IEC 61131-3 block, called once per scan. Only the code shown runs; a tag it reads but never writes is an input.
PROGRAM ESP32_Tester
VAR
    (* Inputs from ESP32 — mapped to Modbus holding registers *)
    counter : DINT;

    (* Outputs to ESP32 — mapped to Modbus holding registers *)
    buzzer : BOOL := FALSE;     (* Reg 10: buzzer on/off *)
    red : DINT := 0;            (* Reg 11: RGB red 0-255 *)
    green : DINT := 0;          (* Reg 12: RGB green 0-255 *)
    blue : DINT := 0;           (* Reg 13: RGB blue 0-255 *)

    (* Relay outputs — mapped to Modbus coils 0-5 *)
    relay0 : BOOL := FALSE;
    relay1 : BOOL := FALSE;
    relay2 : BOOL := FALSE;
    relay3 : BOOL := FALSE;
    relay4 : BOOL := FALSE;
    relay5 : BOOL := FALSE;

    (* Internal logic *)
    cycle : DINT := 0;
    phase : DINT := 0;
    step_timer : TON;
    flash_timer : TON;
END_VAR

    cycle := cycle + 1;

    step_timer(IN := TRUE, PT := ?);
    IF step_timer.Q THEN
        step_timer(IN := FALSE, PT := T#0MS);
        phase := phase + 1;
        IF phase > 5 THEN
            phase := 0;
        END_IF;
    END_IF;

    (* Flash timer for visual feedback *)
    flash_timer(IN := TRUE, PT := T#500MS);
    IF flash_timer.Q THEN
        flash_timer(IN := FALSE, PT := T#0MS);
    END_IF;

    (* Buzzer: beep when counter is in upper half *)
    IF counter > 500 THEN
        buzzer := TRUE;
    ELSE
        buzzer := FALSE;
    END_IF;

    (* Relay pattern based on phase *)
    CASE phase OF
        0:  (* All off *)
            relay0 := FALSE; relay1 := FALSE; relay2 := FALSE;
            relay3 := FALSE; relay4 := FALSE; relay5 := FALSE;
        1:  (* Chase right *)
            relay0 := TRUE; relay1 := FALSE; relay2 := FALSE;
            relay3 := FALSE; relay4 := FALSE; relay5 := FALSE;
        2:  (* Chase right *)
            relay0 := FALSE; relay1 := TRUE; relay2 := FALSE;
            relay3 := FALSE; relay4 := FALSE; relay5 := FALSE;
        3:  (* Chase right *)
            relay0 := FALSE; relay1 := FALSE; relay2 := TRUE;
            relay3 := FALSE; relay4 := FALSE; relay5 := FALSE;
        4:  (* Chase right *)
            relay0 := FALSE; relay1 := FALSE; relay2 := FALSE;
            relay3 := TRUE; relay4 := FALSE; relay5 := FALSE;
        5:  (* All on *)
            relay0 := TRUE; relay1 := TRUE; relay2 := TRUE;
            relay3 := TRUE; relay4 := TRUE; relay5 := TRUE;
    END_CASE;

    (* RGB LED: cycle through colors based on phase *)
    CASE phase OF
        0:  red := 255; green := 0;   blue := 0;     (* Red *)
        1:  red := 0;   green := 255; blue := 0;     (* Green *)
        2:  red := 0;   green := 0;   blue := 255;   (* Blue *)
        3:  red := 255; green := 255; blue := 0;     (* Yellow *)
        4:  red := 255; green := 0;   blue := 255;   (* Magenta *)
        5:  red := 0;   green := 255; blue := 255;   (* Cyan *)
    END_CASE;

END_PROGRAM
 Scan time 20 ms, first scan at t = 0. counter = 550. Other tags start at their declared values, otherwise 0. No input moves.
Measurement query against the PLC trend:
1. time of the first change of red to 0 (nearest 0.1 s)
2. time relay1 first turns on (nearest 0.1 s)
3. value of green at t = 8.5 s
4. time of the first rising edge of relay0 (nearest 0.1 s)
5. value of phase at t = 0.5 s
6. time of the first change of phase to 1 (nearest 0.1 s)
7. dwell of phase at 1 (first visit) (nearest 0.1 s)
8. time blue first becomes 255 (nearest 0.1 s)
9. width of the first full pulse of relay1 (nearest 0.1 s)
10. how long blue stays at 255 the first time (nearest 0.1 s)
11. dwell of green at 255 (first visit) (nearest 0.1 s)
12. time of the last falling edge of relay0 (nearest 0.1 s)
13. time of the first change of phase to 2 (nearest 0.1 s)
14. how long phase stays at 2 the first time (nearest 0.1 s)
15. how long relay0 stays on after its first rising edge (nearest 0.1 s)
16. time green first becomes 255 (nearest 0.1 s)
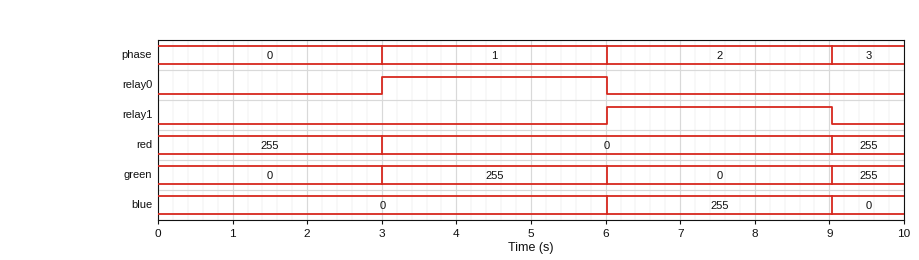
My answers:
3.0 s
6.0 s
0
3.0 s
0
3.0 s
3.0 s
6.0 s
3.0 s
3.0 s
3.0 s
6.0 s
6.0 s
3.0 s
3.0 s
3.0 s
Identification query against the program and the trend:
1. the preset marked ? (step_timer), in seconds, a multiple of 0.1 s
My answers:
3.0 s
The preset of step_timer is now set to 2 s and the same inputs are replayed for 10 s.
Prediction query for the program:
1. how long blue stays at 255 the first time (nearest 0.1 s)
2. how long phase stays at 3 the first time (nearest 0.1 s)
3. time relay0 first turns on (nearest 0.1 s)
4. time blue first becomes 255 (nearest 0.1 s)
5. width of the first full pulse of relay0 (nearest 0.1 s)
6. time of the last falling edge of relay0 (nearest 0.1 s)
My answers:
2.0 s
2.0 s
2.0 s
4.0 s
2.0 s
4.0 s
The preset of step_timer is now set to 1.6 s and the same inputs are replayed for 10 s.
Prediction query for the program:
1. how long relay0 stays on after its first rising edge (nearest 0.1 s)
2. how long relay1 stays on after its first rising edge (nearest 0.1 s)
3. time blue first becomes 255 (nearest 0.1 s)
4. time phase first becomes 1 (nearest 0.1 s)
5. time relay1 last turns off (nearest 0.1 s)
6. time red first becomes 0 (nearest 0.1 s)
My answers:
1.6 s
1.6 s
3.2 s
1.6 s
9.7 s
1.6 s
